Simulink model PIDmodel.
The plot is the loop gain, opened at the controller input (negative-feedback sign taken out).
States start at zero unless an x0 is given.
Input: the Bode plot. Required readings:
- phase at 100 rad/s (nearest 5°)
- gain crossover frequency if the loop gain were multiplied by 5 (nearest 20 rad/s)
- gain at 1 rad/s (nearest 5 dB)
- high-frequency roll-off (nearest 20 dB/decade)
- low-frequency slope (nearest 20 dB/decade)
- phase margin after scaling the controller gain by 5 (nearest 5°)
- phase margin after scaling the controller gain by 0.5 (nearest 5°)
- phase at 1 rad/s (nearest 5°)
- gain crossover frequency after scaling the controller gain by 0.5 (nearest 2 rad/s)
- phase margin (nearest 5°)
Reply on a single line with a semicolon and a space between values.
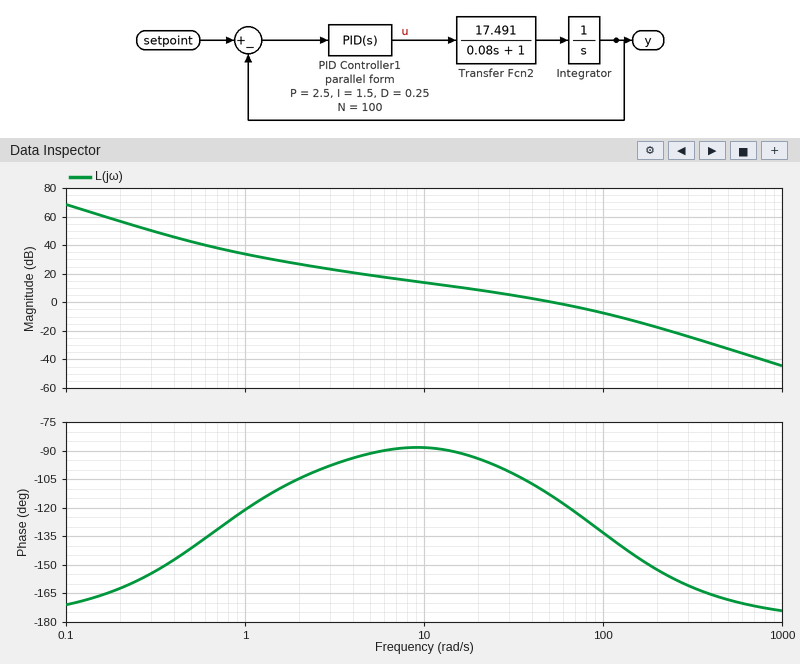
-135°; 160 rad/s; 35 dB; -40 dB/decade; -40 dB/decade; 35°; 80°; -120°; 28 rad/s; 65°
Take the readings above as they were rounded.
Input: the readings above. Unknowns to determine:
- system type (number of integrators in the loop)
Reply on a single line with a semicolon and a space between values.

2
